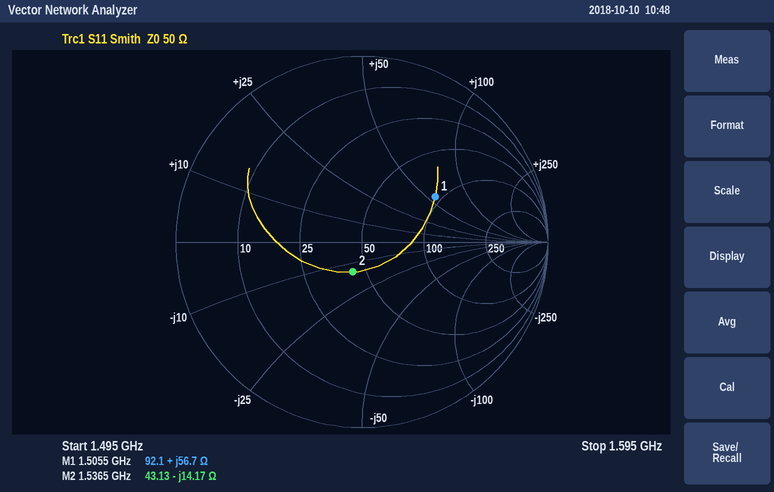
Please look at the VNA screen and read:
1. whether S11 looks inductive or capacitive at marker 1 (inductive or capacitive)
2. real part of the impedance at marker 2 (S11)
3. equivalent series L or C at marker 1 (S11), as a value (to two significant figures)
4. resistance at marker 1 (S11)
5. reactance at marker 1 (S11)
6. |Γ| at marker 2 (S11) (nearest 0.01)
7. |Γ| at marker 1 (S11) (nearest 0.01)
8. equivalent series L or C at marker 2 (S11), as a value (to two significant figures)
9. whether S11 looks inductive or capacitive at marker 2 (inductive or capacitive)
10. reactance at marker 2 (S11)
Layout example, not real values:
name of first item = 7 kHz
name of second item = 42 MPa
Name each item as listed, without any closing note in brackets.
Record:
whether S11 looks inductive or capacitive at marker 1 = inductive
real part of the impedance at marker 2 = 43.13 Ω
equivalent series L or C at marker 1 (S11), as a value = 6.0 nH
resistance at marker 1 = 92.1 Ω
reactance at marker 1 = +56.7 Ω
|Γ| at marker 2 (S11) = 0.17
|Γ| at marker 1 (S11) = 0.46
equivalent series L or C at marker 2 (S11), as a value = 7.3 pF
whether S11 looks inductive or capacitive at marker 2 = capacitive
reactance at marker 2 = -14.17 Ω
